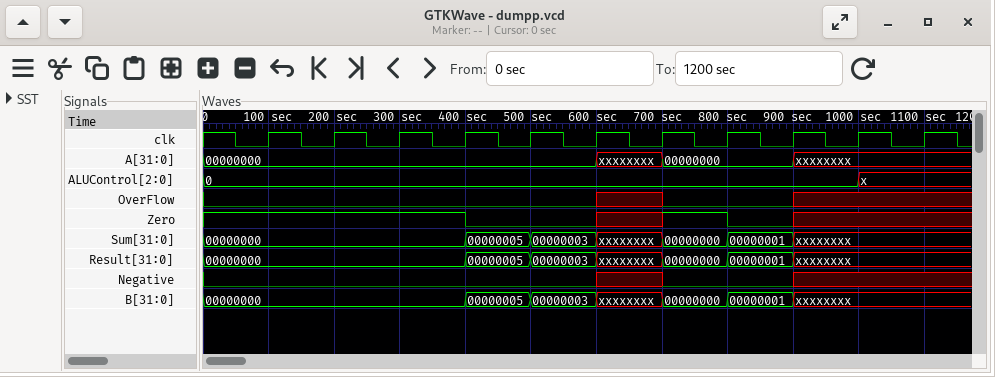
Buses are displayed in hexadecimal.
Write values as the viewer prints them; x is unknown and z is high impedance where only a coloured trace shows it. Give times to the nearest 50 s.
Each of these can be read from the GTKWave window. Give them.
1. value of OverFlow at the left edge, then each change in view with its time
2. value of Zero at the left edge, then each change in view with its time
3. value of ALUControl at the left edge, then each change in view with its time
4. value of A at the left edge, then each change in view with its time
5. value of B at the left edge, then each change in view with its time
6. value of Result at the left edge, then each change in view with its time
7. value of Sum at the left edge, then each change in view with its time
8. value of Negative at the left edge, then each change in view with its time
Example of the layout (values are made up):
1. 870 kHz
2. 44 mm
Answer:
1. 0, x at 600 s, 0 at 700 s, x at 900 s
2. 1, 0 at 400 s, x at 600 s, 1 at 700 s, 0 at 800 s, x at 900 s
3. 0, x at 1000 s
4. 00000000, xxxxxxxx at 600 s, 00000000 at 700 s, xxxxxxxx at 900 s
5. 00000000, 00000005 at 400 s, 00000003 at 500 s, xxxxxxxx at 600 s, 00000000 at 700 s, 00000001 at 800 s, xxxxxxxx at 900 s
6. 00000000, 00000005 at 400 s, 00000003 at 500 s, xxxxxxxx at 600 s, 00000000 at 700 s, 00000001 at 800 s, xxxxxxxx at 900 s
7. 00000000, 00000005 at 400 s, 00000003 at 500 s, xxxxxxxx at 600 s, 00000000 at 700 s, 00000001 at 800 s, xxxxxxxx at 900 s
8. 0, x at 600 s, 0 at 700 s, x at 900 s
